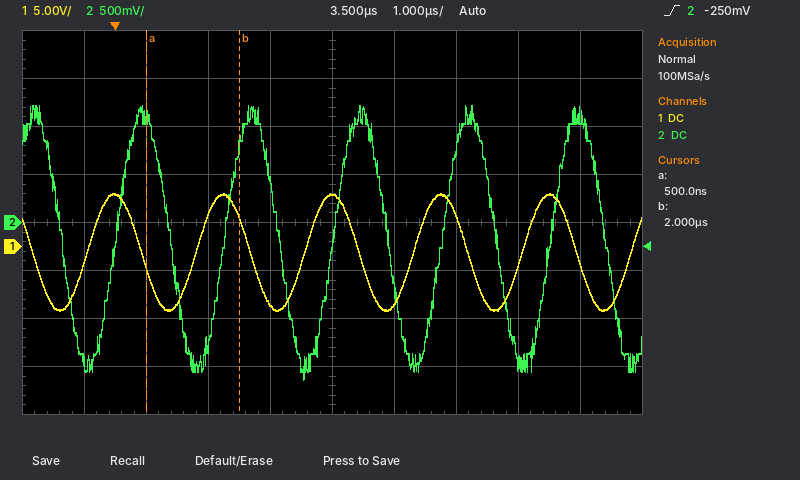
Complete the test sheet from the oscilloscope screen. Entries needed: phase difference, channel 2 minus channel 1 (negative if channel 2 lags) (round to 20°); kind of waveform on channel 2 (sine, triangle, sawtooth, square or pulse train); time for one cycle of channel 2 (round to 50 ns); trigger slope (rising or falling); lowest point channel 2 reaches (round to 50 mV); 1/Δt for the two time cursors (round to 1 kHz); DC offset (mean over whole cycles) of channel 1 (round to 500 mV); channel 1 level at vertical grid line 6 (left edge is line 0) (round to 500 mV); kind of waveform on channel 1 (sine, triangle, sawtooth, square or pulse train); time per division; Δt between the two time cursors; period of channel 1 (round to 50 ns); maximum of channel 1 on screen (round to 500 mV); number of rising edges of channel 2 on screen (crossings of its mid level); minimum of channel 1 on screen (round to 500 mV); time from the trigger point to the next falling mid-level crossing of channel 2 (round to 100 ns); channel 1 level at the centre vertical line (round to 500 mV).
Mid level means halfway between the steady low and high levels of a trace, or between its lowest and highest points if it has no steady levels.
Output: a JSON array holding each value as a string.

["-100°", "sine", "1.75 µs", "rising", "-1.65 V", "667 kHz", "-500 mV", "-6.0 V", "sine", "1 µs", "1.5 µs", "1.75 µs", "5.5 V", "5", "-6.5 V", "900 ns", "5.5 V"]
